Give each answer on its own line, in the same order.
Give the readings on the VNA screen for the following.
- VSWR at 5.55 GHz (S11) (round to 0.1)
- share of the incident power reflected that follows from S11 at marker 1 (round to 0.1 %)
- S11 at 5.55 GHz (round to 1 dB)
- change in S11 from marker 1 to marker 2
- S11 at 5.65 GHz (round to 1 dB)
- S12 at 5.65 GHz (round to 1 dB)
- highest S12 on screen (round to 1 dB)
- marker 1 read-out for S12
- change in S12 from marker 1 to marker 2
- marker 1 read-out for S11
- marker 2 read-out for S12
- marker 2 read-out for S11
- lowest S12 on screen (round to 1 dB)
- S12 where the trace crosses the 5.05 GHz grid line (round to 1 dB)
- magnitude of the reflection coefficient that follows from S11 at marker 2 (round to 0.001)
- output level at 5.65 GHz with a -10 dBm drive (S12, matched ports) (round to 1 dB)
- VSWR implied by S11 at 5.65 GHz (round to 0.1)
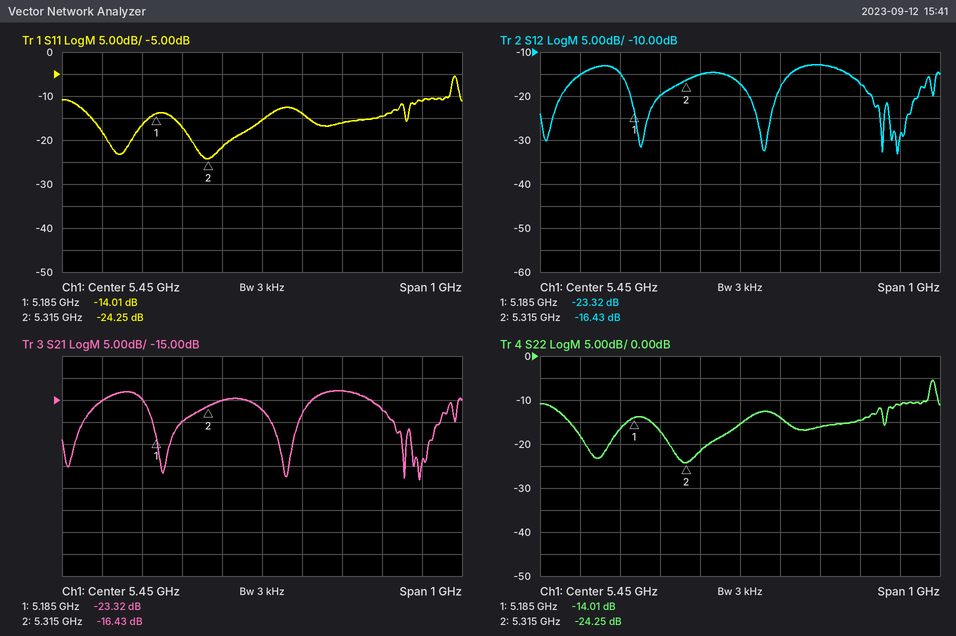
1.5
4.0 %
-14 dB
-10.24 dB
-16 dB
-13 dB
-13 dB
-23.32 dB
6.89 dB
-14.01 dB
-16.43 dB
-24.25 dB
-33 dB
-15 dB
0.061
-23 dBm
1.4
